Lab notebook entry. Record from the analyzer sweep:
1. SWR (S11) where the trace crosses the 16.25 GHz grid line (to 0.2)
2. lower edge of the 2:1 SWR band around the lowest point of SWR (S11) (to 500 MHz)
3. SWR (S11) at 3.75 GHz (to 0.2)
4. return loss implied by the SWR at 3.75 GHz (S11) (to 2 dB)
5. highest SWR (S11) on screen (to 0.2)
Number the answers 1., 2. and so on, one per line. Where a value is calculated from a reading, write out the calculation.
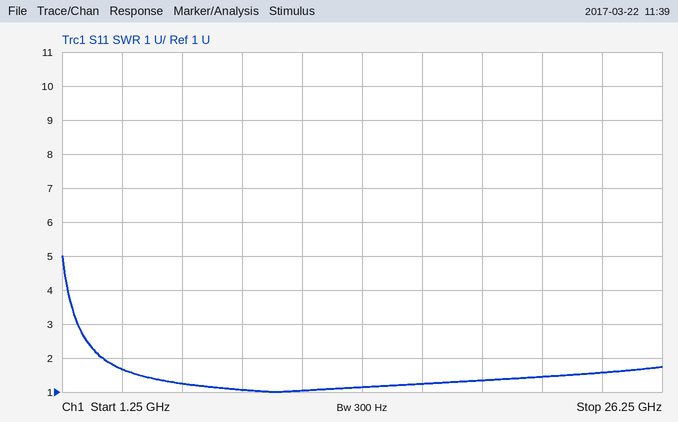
1. 1.2
2. 3.0 GHz
3. 1.6
4. −20 log10((1.6 − 1)/(1.6 + 1)) ≈ 12.7 dB, so 12 dB to the nearest 2 dB
5. 5.0
